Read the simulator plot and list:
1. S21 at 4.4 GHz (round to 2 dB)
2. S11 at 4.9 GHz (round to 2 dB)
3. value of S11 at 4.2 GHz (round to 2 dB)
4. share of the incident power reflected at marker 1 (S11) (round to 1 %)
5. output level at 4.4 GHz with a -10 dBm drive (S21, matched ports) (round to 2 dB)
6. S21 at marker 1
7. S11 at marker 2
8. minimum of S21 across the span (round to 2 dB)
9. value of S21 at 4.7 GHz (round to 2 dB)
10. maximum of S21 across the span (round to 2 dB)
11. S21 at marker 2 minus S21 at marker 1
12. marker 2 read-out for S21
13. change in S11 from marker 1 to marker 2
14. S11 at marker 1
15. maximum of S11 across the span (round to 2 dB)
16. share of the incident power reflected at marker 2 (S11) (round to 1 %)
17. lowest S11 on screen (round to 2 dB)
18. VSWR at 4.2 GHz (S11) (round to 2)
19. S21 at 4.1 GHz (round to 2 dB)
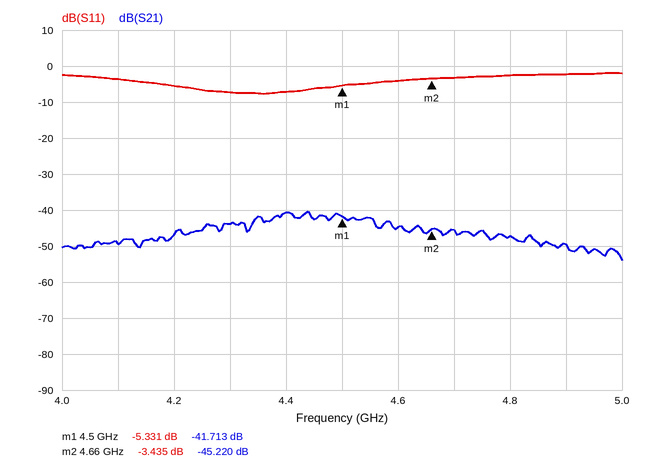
-40 dB
-2 dB
-6 dB
29 %
-50 dBm
-41.713 dB
-3.435 dB
-54 dB
-46 dB
-40 dB
-3.507 dB
-45.220 dB
1.896 dB
-5.331 dB
-2 dB
45 %
-8 dB
4
-50 dB
